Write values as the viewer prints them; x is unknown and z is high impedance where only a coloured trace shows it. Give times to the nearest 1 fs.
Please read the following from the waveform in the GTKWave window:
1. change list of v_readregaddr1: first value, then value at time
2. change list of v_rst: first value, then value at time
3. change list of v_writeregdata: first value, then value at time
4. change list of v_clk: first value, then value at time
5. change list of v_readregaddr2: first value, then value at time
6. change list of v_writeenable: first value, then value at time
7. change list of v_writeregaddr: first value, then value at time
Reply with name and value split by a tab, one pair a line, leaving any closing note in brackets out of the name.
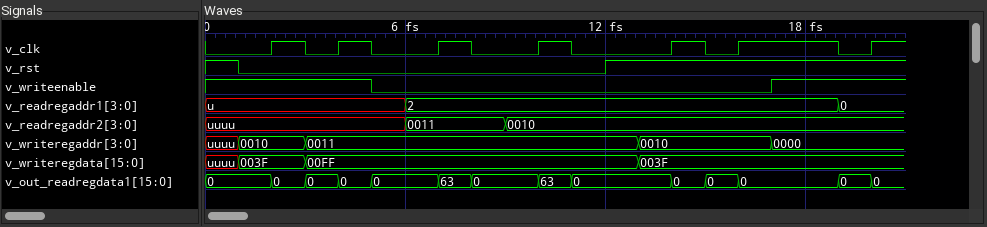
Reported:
change list of v_readregaddr1: first value, then value at time	u, 2 at 6 fs, 0 at 19 fs
change list of v_rst: first value, then value at time	1, 0 at 1 fs, 1 at 12 fs
change list of v_writeregdata: first value, then value at time	uuuu, 003F at 1 fs, 00FF at 3 fs, 003F at 13 fs
change list of v_clk: first value, then value at time	0, 1 at 2 fs, 0 at 3 fs, 1 at 4 fs, 0 at 5 fs, 1 at 7 fs, 0 at 8 fs, 1 at 10 fs, 0 at 11 fs, 1 at 14 fs, 0 at 15 fs, 1 at 16 fs, 0 at 19 fs, 1 at 20 fs
change list of v_readregaddr2: first value, then value at time	uuuu, 0011 at 6 fs, 0010 at 9 fs
change list of v_writeenable: first value, then value at time	1, 0 at 5 fs, 1 at 17 fs
change list of v_writeregaddr: first value, then value at time	uuuu, 0010 at 1 fs, 0011 at 3 fs, 0010 at 13 fs, 0000 at 17 fs
